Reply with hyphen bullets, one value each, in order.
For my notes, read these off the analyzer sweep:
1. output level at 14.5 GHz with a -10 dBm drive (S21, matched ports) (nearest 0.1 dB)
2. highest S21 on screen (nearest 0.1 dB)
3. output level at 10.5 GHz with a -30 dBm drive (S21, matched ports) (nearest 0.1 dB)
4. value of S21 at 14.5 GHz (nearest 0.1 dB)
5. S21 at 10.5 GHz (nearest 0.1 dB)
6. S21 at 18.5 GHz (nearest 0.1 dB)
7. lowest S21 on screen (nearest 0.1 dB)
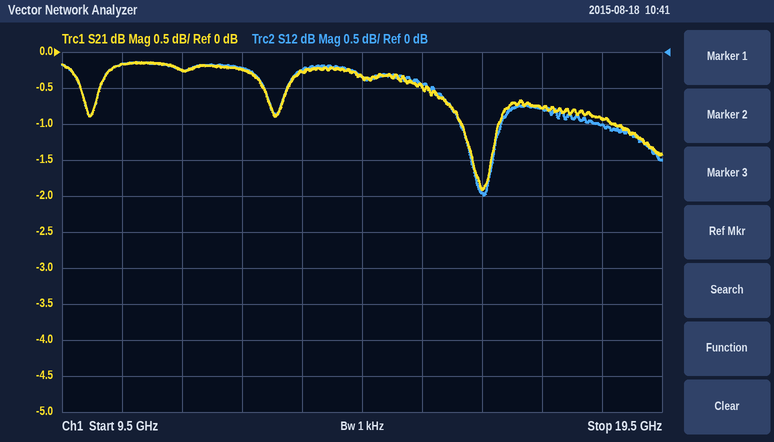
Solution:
- -10.3 dBm
- -0.1 dB
- -30.2 dBm
- -0.3 dB
- -0.2 dB
- -0.9 dB
- -1.9 dB
